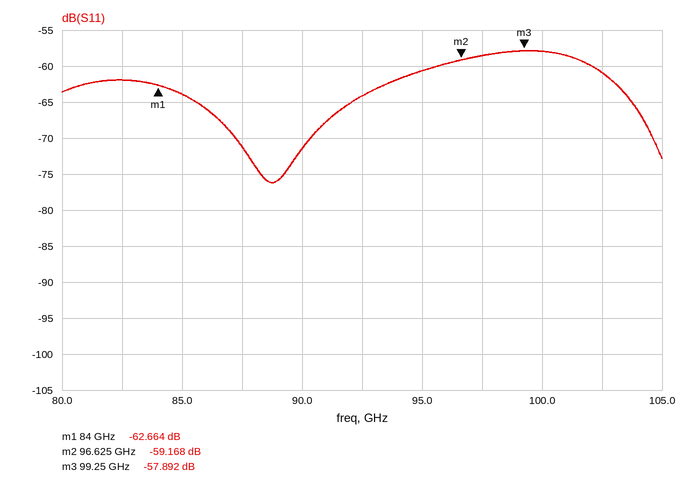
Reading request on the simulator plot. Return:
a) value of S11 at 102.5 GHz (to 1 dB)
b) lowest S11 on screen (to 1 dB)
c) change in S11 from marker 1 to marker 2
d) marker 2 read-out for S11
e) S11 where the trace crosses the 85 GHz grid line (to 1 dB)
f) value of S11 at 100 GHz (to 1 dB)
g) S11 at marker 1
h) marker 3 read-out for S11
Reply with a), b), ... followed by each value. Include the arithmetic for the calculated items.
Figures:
a) -61 dB
b) -76 dB
c) -59.168 − (-62.664) = 3.496 dB
d) -59.168 dB
e) -64 dB
f) -58 dB
g) -62.664 dB
h) -57.892 dB
